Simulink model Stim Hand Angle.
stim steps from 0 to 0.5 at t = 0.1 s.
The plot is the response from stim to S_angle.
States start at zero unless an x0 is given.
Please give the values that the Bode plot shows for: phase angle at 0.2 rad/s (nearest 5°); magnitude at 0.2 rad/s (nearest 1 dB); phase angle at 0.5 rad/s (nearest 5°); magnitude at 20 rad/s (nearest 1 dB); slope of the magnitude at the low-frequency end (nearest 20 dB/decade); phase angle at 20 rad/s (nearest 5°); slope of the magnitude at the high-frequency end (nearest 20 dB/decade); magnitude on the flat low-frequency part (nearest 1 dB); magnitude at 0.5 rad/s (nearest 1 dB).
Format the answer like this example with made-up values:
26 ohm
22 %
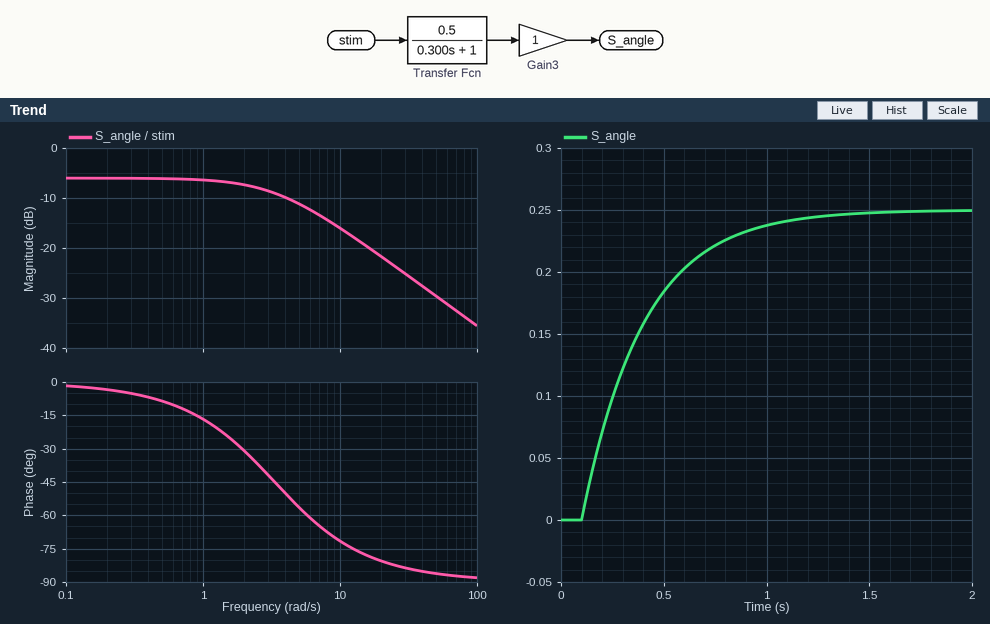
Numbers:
-5°
-6 dB
-10°
-22 dB
0 dB/decade
-80°
-20 dB/decade
-6 dB
-6 dB
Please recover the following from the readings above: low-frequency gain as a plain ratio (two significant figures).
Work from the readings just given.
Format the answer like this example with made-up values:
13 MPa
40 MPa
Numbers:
0.50
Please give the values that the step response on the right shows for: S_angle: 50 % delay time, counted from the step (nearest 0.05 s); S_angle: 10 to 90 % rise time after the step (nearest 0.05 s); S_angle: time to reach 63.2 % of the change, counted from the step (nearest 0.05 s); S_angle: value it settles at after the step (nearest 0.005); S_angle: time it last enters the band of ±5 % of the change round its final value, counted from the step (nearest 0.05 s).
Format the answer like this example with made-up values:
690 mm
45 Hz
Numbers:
0.20 s
0.65 s
0.30 s
0.250
0.90 s
